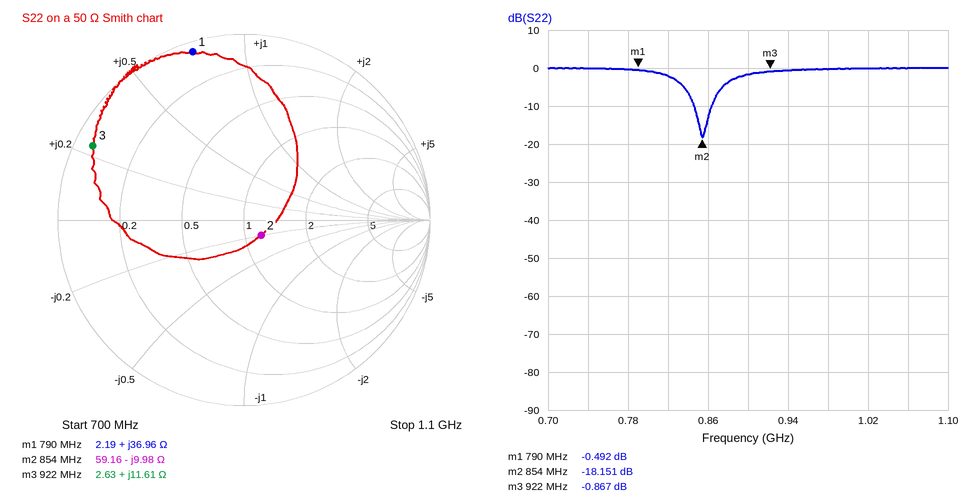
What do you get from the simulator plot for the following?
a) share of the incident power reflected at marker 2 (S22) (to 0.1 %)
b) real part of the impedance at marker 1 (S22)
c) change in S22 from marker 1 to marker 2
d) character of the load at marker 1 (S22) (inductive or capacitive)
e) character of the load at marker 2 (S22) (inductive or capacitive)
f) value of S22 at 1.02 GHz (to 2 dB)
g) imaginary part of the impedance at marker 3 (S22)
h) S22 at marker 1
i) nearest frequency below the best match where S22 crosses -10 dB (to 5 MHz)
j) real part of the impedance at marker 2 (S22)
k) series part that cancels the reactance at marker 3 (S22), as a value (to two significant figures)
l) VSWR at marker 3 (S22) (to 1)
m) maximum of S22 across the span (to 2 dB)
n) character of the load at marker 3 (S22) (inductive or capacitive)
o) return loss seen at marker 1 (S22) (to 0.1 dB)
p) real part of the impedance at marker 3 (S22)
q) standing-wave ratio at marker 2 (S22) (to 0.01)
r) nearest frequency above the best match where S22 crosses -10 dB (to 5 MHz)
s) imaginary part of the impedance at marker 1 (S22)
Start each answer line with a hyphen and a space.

- 1.5 %
- 2.19 Ω
- -17.659 dB
- inductive
- capacitive
- 0 dB
- +11.61 Ω
- -0.492 dB
- 845 MHz
- 59.16 Ω
- 15 pF
- 20
- 0 dB
- inductive
- 0.5 dB
- 2.63 Ω
- 1.28
- 865 MHz
- +36.96 Ω
